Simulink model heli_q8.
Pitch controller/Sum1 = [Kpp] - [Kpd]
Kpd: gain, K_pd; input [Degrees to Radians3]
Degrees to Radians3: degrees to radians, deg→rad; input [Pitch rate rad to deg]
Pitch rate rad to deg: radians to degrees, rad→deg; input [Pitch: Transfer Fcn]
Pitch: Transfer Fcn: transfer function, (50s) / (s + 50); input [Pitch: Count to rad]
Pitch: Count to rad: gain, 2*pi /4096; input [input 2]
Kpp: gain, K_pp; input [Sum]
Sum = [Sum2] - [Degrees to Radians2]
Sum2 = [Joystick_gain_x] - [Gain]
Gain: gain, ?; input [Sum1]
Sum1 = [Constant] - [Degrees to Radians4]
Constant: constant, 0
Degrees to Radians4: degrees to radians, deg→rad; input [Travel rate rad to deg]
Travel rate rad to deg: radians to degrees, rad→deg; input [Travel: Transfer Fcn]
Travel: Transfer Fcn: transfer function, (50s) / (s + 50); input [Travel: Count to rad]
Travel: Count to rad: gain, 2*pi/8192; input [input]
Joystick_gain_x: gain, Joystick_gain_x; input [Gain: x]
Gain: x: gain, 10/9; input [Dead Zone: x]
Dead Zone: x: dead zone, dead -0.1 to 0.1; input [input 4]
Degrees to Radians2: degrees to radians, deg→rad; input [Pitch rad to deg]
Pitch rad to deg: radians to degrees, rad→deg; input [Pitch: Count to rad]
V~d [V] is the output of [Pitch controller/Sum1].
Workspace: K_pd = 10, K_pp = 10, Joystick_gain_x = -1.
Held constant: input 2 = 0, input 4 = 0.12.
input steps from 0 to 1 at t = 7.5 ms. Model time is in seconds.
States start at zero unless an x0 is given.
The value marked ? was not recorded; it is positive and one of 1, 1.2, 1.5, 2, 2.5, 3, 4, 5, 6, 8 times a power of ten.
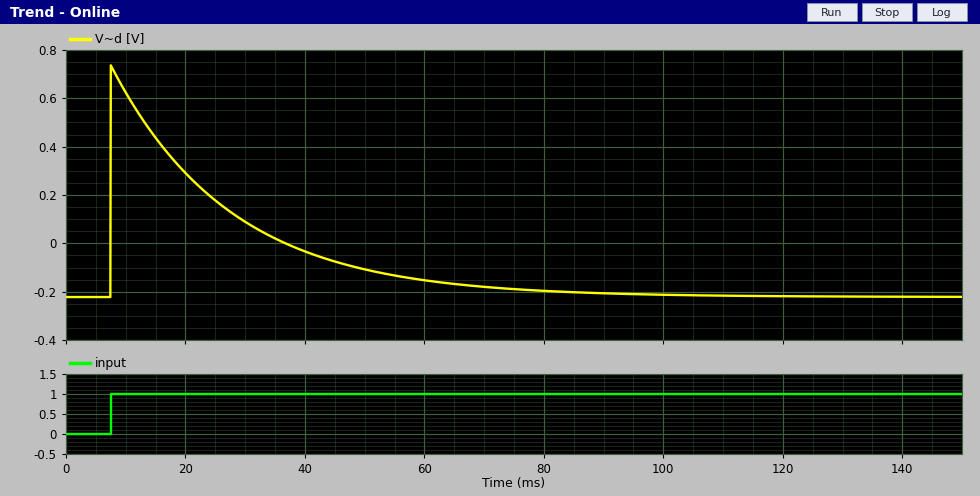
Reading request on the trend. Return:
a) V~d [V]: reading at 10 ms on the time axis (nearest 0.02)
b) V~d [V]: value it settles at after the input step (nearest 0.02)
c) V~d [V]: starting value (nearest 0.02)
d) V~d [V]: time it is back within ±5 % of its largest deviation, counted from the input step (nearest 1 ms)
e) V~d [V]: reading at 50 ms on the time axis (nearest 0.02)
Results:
0.62
-0.22
-0.22
60 ms
-0.10
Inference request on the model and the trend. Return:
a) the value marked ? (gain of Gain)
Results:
2.5
